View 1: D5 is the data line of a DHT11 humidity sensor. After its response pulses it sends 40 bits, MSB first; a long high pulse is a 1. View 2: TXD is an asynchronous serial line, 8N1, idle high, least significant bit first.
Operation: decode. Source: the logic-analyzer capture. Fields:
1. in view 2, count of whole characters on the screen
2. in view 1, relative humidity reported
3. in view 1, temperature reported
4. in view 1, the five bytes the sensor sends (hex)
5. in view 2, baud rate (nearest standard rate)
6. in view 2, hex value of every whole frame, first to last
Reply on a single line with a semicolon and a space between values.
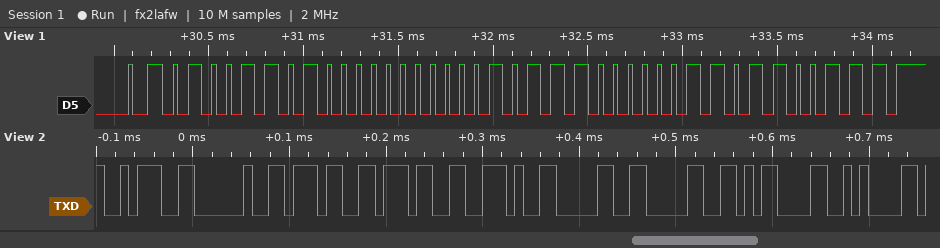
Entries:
9; 77 %; 23.3 °C; 4D 00 17 03 67; 115200 baud; 3A 20 37 37 2E 30 30 0D 0A
